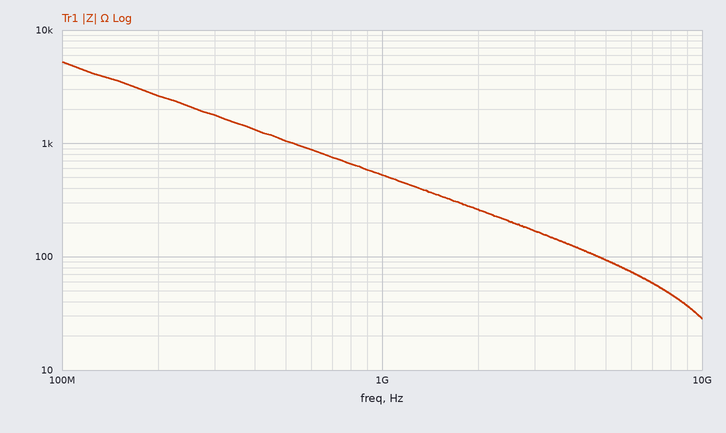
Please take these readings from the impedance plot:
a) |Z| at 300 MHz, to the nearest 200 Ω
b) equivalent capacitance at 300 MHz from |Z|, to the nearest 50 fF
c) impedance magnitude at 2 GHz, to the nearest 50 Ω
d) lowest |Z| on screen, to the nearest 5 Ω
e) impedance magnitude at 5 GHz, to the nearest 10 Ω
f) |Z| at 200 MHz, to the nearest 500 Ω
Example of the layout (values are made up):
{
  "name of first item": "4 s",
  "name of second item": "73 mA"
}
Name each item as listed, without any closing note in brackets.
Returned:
{
  "|Z| at 300 MHz, to the nearest 200 Ω": "1.8 kΩ",
  "equivalent capacitance at 300 MHz from |Z|, to the nearest 50 fF": "300 fF",
  "impedance magnitude at 2 GHz, to the nearest 50 Ω": "250 Ω",
  "lowest |Z| on screen, to the nearest 5 Ω": "30 Ω",
  "impedance magnitude at 5 GHz, to the nearest 10 Ω": "90 Ω",
  "|Z| at 200 MHz, to the nearest 500 Ω": "2.5 kΩ"
}
